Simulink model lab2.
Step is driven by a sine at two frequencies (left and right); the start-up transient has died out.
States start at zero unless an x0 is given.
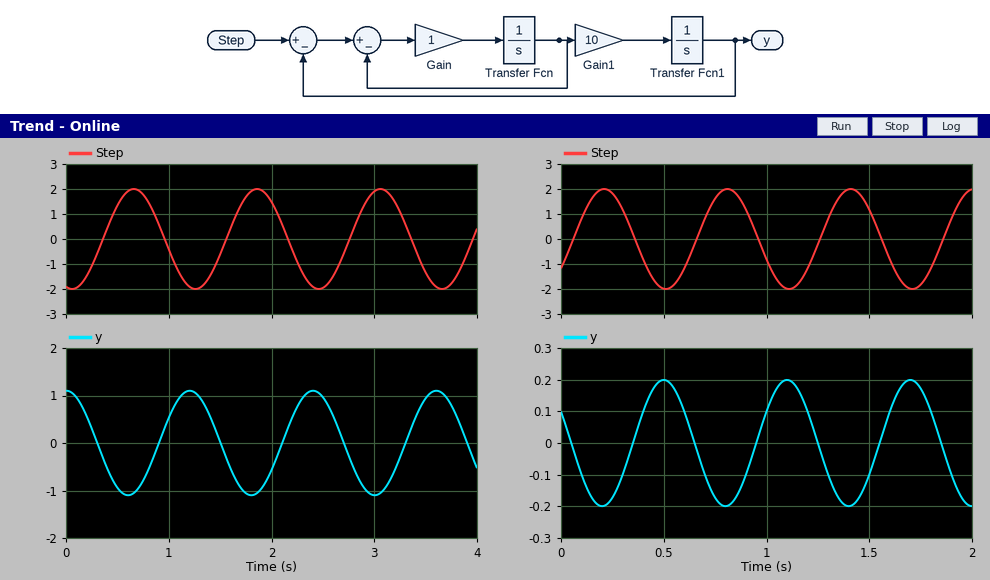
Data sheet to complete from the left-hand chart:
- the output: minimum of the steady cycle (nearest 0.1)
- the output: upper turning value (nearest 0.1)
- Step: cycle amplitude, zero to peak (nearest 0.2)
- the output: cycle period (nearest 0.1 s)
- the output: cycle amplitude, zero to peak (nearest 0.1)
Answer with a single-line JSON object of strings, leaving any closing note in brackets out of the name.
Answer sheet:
{"the output: minimum of the steady cycle": "-1.1", "the output: upper turning value": "1.1", "Step: cycle amplitude, zero to peak": "2.0", "the output: cycle period": "1.2 s", "the output: cycle amplitude, zero to peak": "1.1"}
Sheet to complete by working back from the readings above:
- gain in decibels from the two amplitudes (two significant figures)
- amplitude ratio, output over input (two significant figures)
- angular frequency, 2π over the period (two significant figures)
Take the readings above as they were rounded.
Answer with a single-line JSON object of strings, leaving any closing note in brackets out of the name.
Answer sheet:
{"gain in decibels from the two amplitudes": "-5.2 dB", "amplitude ratio, output over input": "0.55", "angular frequency, 2π over the period": "5.2 rad/s"}
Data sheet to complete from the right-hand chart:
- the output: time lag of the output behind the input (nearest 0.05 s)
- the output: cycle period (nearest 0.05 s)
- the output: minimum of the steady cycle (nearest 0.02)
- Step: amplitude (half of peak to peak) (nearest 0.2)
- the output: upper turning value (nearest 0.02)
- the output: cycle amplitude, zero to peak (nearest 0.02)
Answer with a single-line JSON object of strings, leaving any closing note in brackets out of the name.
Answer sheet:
{"the output: time lag of the output behind the input": "0.30 s", "the output: cycle period": "0.60 s", "the output: minimum of the steady cycle": "-0.20", "Step: amplitude (half of peak to peak)": "2.0", "the output: upper turning value": "0.20", "the output: cycle amplitude, zero to peak": "0.20"}
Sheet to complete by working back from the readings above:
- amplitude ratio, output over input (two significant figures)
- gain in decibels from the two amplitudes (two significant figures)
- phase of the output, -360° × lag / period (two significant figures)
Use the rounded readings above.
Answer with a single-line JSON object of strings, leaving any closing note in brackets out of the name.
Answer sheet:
{"amplitude ratio, output over input": "0.10", "gain in decibels from the two amplitudes": "-20 dB", "phase of the output, -360° × lag / period": "-180°"}
